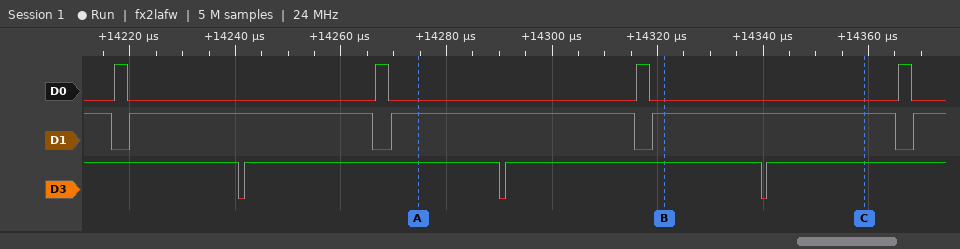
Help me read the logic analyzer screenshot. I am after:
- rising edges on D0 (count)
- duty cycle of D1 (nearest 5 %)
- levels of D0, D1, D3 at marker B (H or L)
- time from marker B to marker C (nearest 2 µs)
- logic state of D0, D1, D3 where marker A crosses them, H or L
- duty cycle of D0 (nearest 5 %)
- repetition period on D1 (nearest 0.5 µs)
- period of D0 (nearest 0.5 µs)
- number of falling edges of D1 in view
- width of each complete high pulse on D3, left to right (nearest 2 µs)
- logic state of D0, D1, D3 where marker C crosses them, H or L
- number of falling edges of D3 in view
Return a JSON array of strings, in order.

["4", "95 %", "D0=L, D1=H, D3=H", "38 µs", "D0=L, D1=H, D3=H", "5 %", "49.5 µs", "49.5 µs", "4", "48 µs, 48 µs", "D0=L, D1=H, D3=H", "3"]
